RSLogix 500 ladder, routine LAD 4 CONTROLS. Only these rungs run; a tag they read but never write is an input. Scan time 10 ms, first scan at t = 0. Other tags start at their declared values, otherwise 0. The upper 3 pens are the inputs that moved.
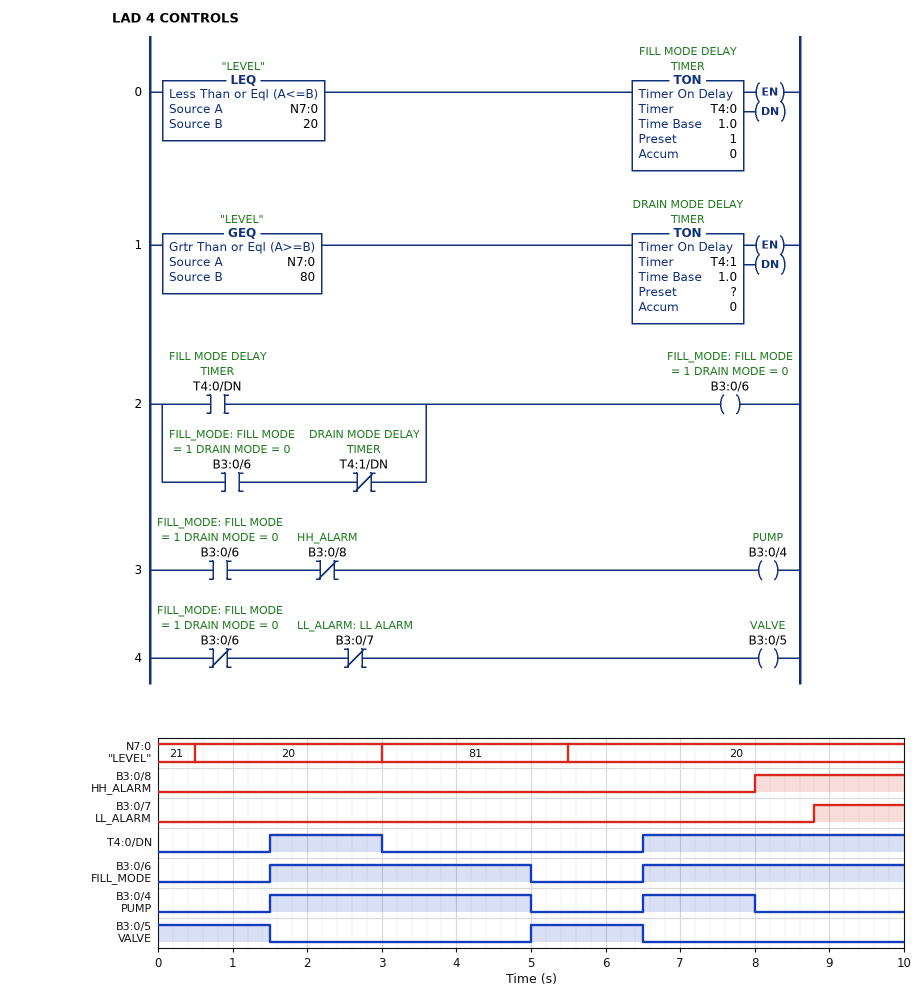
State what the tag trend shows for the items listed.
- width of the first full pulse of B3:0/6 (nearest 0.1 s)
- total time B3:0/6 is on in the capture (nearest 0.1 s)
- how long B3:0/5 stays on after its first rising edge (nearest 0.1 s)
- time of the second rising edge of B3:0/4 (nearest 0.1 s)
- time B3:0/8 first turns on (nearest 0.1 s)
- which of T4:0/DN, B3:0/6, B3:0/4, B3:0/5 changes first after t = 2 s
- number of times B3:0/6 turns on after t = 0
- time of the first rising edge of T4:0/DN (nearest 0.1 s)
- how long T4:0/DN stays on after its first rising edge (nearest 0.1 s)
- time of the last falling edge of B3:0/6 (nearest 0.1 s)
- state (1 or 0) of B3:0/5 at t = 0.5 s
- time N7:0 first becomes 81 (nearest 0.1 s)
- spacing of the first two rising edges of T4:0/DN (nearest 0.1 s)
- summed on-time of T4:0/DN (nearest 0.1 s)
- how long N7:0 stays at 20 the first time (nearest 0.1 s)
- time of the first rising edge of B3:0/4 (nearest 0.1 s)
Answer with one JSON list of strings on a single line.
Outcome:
["3.5 s", "7.0 s", "1.5 s", "6.5 s", "8.0 s", "T4:0/DN", "2", "1.5 s", "1.5 s", "5.0 s", "1", "3.0 s", "5.0 s", "5.0 s", "2.5 s", "1.5 s"]
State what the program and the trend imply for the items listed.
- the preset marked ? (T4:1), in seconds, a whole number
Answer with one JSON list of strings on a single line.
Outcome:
["2 s"]
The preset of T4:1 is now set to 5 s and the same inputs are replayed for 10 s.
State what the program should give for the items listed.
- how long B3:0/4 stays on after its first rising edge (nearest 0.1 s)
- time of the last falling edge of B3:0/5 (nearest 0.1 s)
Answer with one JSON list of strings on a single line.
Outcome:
["6.5 s", "1.5 s"]
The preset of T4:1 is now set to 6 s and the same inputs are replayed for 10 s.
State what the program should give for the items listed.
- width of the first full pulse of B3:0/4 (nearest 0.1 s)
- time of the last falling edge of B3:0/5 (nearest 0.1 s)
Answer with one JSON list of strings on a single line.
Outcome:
["6.5 s", "1.5 s"]
